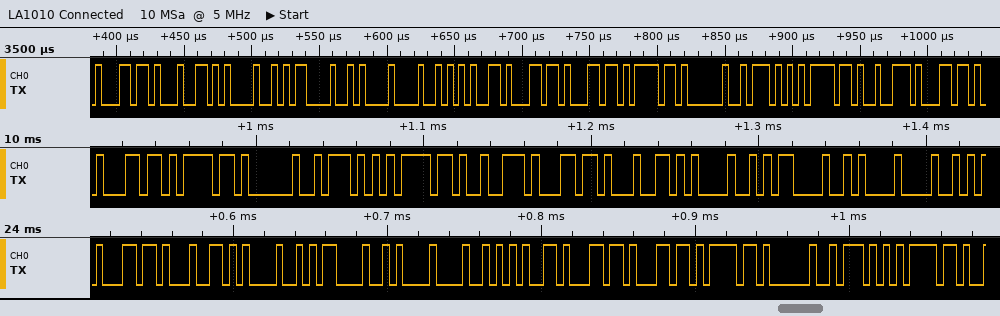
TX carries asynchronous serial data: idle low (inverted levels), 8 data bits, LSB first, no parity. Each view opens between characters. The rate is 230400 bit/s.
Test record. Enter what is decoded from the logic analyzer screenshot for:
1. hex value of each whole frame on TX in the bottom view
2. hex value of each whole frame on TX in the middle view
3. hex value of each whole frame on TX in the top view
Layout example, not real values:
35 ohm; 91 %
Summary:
27, 37, BD, E5, EB, 6F, 35, 27, 27, 21, BF, 51, 21; 27, 21, BF, 51, 21, 1B, 27, 37, BD, E5, EB, 6F; 27, 37, BD, E5, EB, 6F, 35, 27, 27, 21, BF, 51, 21, 1B, 27
